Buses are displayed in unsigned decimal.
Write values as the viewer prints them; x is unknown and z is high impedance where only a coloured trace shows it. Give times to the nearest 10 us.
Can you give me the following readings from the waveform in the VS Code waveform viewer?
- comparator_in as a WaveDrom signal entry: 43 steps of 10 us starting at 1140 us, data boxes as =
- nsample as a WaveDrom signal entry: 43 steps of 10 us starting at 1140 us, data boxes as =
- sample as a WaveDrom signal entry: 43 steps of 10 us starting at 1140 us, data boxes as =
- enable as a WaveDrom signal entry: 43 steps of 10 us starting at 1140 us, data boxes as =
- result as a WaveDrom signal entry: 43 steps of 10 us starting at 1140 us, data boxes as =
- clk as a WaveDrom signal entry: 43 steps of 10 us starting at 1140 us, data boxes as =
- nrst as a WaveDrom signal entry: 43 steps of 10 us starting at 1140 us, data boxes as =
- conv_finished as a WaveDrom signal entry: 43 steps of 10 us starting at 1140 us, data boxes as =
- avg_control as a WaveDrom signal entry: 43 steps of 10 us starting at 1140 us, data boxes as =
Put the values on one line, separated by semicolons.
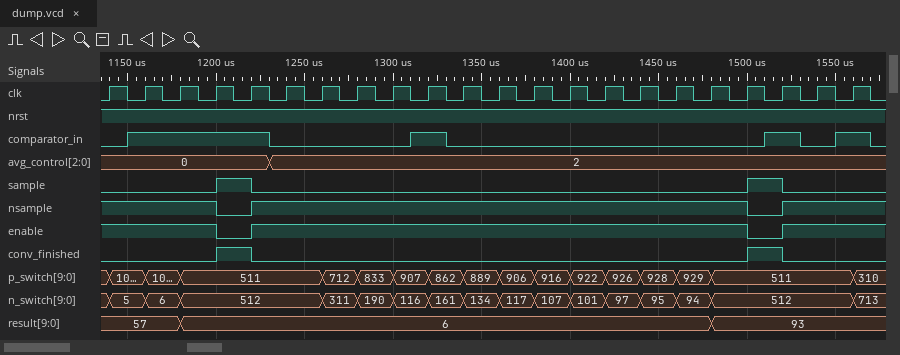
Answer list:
{name: 'comparator_in', wave: '01.......0.......1.0.................1.0.1.'}; {name: 'nsample', wave: '1.....0.1...........................0.1....'}; {name: 'sample', wave: '0.....1.0...........................1.0....'}; {name: 'enable', wave: '1.....0.1...........................0.1....'}; {name: 'result', wave: '=...=.............................=........', data: '57 6 93'}; {name: 'clk', wave: '1010101010101010101010101010101010101010101'}; {name: 'nrst', wave: '1..........................................'}; {name: 'conv_finished', wave: '0.....1.0...........................1.0....'}; {name: 'avg_control', wave: '=........=.................................', data: '0 2'}
